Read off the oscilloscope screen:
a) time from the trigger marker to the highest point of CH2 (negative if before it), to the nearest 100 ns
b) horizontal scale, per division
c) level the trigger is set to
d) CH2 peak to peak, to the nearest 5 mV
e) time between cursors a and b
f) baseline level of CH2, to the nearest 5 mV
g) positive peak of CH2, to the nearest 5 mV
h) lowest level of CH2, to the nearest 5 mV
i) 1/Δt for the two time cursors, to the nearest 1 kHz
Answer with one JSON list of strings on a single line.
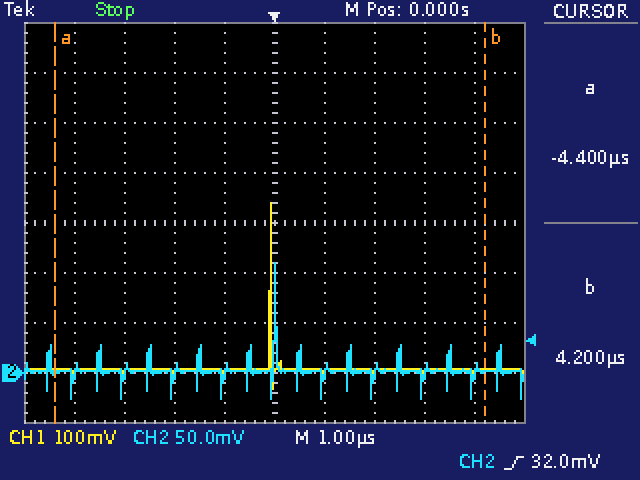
["0.0 µs", "1 µs", "32.0 mV", "135 mV", "8.6 µs", "0 mV", "110 mV", "-25 mV", "116 kHz"]
